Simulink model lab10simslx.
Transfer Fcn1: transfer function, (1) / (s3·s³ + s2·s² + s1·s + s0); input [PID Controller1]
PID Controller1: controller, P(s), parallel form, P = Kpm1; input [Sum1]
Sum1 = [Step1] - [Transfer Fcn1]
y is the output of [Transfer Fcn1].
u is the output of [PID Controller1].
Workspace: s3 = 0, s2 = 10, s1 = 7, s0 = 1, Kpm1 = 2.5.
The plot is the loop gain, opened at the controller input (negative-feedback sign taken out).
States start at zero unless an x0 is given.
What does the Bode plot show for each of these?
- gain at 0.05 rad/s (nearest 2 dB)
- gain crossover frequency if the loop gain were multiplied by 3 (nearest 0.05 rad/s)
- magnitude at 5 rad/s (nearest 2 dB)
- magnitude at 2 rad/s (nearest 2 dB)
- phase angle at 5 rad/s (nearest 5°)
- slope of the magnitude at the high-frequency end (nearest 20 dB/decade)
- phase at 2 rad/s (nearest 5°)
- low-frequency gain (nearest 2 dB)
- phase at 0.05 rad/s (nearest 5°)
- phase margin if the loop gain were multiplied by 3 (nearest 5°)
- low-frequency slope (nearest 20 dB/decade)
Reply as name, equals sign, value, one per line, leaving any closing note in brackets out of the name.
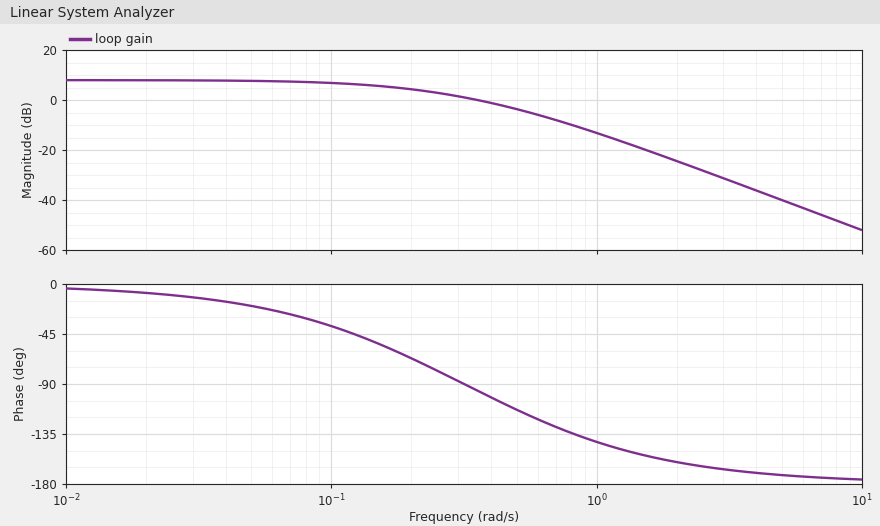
gain at 0.05 rad/s = 8 dB
gain crossover frequency if the loop gain were multiplied by 3 = 0.80 rad/s
magnitude at 5 rad/s = -40 dB
magnitude at 2 rad/s = -24 dB
phase angle at 5 rad/s = -170°
slope of the magnitude at the high-frequency end = -40 dB/decade
phase at 2 rad/s = -160°
low-frequency gain = 8 dB
phase at 0.05 rad/s = -20°
phase margin if the loop gain were multiplied by 3 = 45°
low-frequency slope = 0 dB/decade
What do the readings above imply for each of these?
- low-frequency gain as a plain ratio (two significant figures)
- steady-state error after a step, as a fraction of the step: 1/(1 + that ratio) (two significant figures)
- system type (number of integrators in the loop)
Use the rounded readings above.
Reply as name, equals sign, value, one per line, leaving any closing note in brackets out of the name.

low-frequency gain as a plain ratio = 2.5
steady-state error after a step, as a fraction of the step: 1/(1 + that ratio) = 0.29
system type = 0
